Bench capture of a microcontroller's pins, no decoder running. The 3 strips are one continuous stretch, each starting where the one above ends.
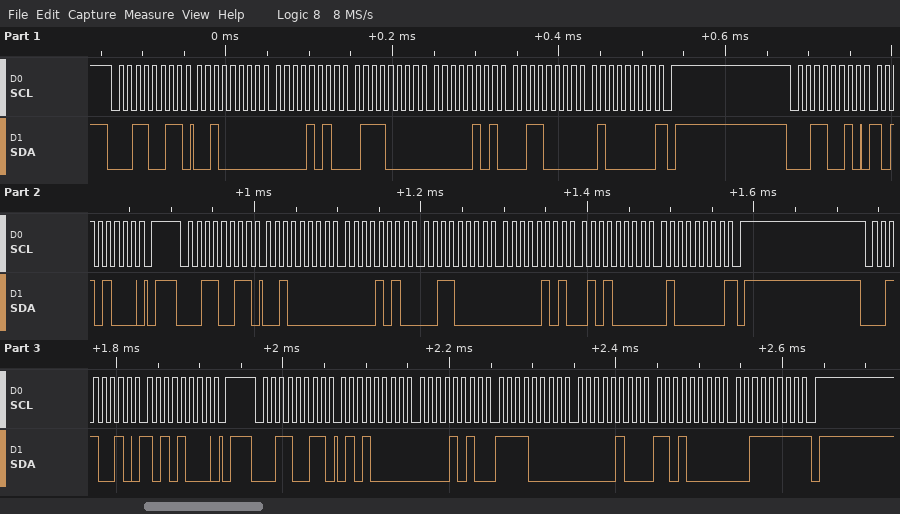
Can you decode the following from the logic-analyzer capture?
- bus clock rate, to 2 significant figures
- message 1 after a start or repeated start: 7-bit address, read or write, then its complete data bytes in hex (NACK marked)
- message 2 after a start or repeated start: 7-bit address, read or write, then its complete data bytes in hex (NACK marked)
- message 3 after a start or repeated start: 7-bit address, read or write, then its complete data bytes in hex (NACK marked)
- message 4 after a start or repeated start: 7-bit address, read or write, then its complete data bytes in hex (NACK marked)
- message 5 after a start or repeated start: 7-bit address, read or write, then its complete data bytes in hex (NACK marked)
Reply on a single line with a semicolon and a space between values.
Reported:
100 kHz; 0x19 read: 20 0A 70 05 30 40 NACK; 0x19 write: A8; 0x19 read: 20 0A 30 05 50 40 NACK; 0x19 write: A8; 0x19 read: 50 0A F0 04 D0 3F NACK
